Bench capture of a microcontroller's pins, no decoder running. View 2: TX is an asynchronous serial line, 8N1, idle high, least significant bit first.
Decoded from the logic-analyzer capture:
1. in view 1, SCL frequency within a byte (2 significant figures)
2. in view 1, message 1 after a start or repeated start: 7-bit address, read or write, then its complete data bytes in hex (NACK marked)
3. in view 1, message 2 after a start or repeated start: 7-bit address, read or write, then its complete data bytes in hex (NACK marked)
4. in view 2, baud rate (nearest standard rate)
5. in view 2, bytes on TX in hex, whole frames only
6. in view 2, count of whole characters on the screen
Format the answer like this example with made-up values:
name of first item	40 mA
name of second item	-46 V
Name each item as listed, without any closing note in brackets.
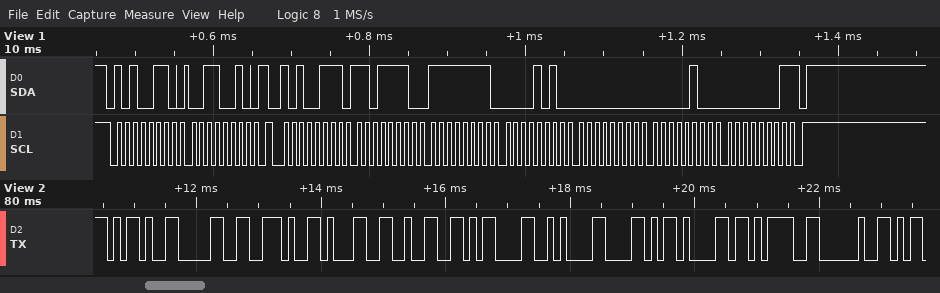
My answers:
in view 1, SCL frequency within a byte	100 kHz
in view 1, message 1 after a start or repeated start: 7-bit address, read or write, then its complete data bytes in hex	0x53 write: 32
in view 1, message 2 after a start or repeated start: 7-bit address, read or write, then its complete data bytes in hex	0x53 read: DE FF 0A 00 04 01 NACK
in view 2, baud rate	9600 baud
in view 2, bytes on TX in hex, whole frames only	2D 30 2E 31 32 0D 0A 58 61 3D 20
in view 2, count of whole characters on the screen	11
